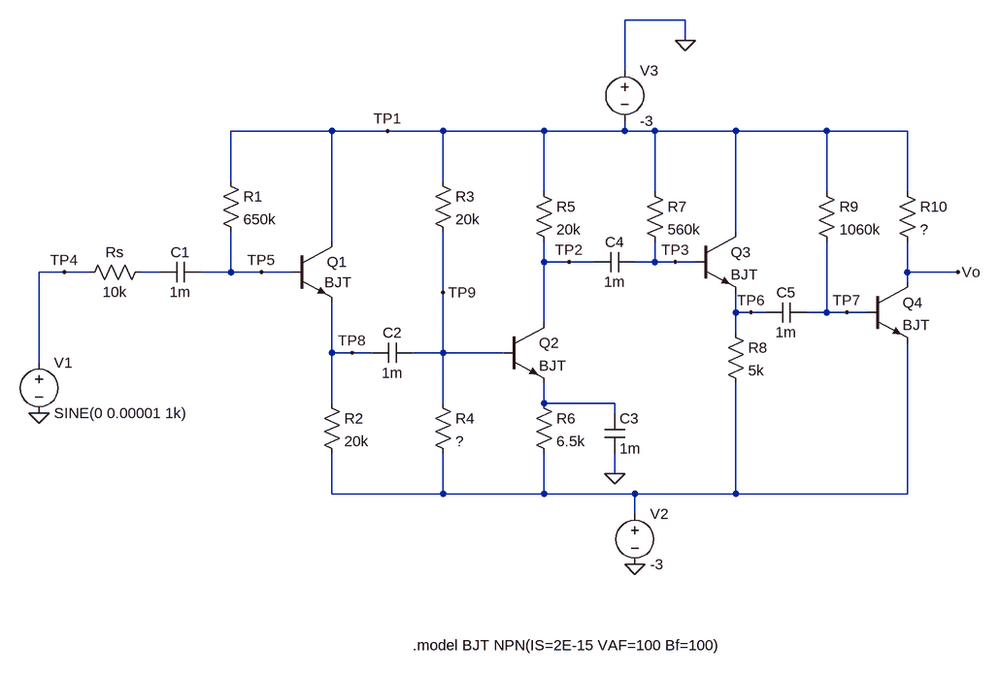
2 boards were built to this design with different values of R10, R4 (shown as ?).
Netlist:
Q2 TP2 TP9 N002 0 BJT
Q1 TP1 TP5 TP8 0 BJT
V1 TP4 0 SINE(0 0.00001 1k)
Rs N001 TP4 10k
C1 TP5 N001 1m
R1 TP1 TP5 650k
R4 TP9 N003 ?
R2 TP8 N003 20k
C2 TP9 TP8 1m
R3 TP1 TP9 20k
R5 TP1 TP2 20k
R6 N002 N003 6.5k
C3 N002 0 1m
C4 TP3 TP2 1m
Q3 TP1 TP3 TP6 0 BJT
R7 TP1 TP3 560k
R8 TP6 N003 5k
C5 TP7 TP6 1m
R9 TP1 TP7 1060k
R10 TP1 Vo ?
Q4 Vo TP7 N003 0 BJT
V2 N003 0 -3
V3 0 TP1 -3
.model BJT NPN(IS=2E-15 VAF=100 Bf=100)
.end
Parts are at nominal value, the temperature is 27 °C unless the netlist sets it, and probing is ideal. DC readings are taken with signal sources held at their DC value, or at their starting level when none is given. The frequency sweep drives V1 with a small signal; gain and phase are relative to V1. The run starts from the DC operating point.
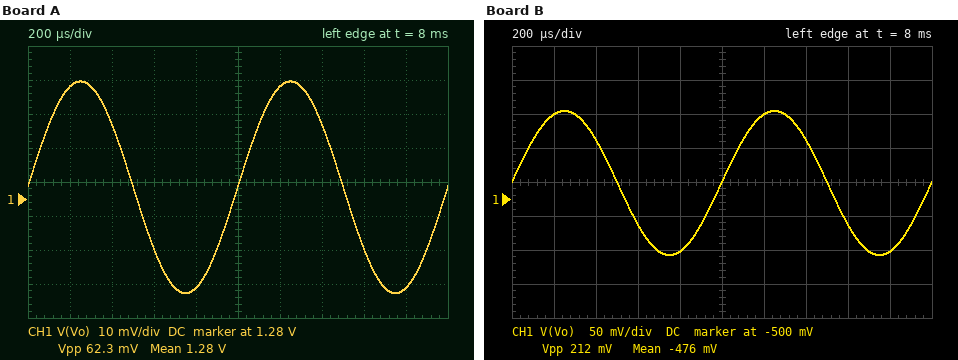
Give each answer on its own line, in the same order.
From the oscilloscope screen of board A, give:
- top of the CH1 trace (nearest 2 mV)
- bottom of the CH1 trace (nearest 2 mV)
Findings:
1.314 V
1.252 V
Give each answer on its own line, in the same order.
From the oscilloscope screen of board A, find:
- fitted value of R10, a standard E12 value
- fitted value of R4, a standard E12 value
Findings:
3.3 kΩ
4.7 kΩ
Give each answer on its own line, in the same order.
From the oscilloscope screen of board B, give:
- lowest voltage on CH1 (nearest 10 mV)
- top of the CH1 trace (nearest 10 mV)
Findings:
-580 mV
-370 mV
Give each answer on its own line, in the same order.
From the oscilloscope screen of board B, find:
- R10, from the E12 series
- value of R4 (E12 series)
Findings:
6.8 kΩ
6.8 kΩ
